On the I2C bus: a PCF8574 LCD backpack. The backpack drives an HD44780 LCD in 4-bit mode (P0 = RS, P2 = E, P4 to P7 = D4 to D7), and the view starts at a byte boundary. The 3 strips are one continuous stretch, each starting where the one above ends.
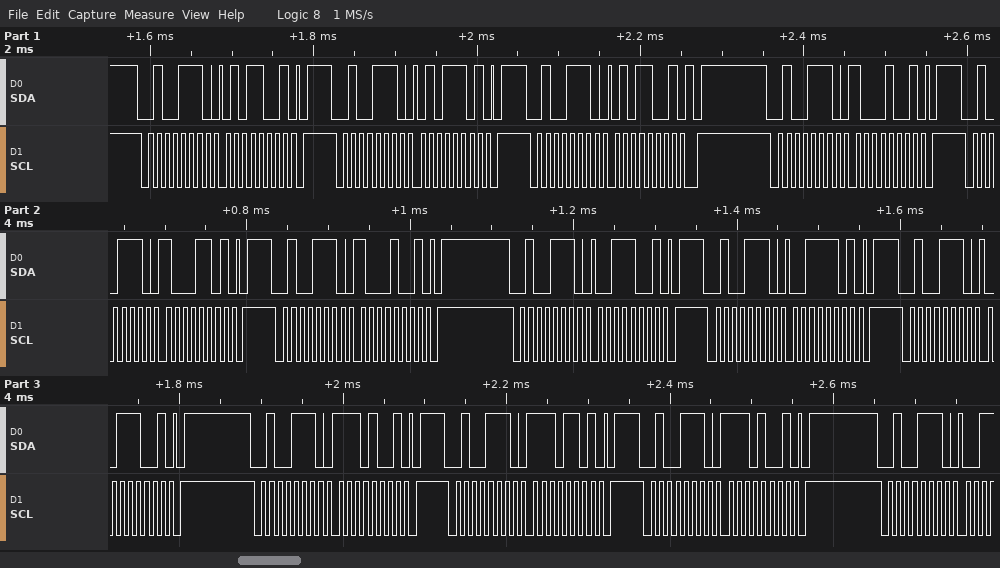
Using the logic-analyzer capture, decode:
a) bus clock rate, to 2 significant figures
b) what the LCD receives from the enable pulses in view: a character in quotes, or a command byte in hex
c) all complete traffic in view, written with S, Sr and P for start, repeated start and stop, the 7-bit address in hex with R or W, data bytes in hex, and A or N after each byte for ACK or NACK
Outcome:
100 kHz
'X' '>'
S 27W A 59 A P S 27W A 5D A P S 27W A 59 A P S 27W A 89 A P S 27W A 8D A P S 27W A 89 A P S 27W A 39 A P S 27W A 3D A P S 27W A 39 A P S 27W A E9 A P S 27W A ED A P S 27W A E9 A P S 27W A
